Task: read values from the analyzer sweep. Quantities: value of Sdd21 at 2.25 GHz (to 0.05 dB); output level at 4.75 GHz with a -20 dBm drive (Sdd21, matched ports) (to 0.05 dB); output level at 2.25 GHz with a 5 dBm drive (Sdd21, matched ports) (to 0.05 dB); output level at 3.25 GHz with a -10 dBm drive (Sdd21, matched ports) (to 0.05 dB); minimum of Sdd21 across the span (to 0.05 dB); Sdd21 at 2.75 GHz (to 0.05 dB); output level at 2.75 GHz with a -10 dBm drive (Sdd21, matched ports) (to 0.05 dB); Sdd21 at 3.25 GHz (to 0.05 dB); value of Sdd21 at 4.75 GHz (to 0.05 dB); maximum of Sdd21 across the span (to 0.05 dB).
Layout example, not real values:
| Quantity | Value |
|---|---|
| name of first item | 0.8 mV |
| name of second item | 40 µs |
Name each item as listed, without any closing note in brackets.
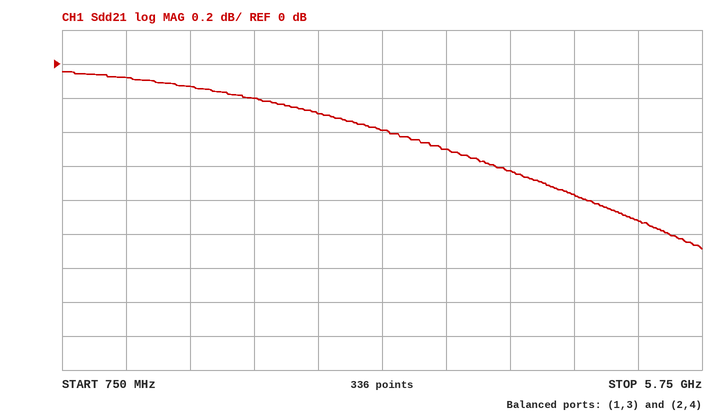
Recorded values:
| Quantity | Value |
|---|---|
| value of Sdd21 at 2.25 GHz | -0.20 dB |
| output level at 4.75 GHz with a -20 dBm drive (Sdd21, matched ports) | -20.75 dBm |
| output level at 2.25 GHz with a 5 dBm drive (Sdd21, matched ports) | 4.80 dBm |
| output level at 3.25 GHz with a -10 dBm drive (Sdd21, matched ports) | -10.40 dBm |
| minimum of Sdd21 across the span | -1.10 dB |
| Sdd21 at 2.75 GHz | -0.30 dB |
| output level at 2.75 GHz with a -10 dBm drive (Sdd21, matched ports) | -10.30 dBm |
| Sdd21 at 3.25 GHz | -0.40 dB |
| value of Sdd21 at 4.75 GHz | -0.75 dB |
| maximum of Sdd21 across the span | -0.05 dB |
